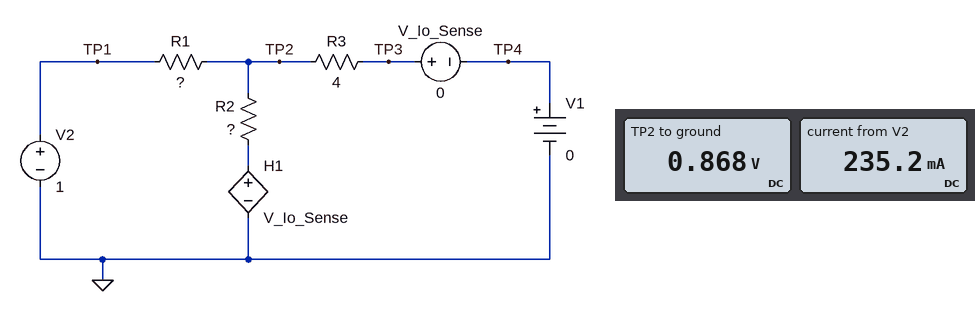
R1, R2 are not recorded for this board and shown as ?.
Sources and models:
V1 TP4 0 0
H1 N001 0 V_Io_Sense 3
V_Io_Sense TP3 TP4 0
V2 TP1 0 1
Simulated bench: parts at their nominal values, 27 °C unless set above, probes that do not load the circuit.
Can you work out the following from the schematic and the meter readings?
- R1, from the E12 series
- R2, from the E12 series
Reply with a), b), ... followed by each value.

a) 0.56 Ω
b) 12 Ω
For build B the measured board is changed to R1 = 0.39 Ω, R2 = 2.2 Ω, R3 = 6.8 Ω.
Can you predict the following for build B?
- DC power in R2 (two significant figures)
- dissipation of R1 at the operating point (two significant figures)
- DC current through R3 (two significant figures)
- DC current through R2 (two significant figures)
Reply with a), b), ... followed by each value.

a) 110 mW
b) 47 mW
c) 130 mA
d) 220 mA
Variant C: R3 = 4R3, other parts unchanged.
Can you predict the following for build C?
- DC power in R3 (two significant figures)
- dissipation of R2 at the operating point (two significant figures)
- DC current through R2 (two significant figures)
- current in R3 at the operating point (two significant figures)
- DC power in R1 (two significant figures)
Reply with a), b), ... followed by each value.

a) 180 mW
b) 5.8 mW
c) 22 mA
d) 200 mA
e) 28 mW
